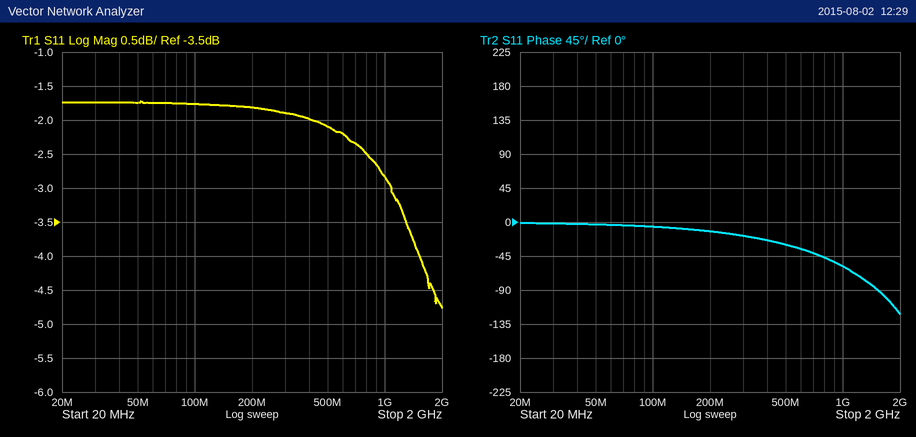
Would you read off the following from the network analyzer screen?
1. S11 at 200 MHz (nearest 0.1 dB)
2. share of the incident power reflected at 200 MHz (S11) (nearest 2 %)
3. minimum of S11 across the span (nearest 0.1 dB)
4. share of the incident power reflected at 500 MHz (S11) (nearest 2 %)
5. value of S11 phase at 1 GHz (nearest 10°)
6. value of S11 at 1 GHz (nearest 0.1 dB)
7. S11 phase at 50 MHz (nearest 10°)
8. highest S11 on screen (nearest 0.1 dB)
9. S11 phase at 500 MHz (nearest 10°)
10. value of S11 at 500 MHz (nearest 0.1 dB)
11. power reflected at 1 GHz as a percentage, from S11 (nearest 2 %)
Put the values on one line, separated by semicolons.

-1.8 dB; 66 %; -4.8 dB; 62 %; -60°; -2.8 dB; 0°; -1.7 dB; -30°; -2.1 dB; 52 %
